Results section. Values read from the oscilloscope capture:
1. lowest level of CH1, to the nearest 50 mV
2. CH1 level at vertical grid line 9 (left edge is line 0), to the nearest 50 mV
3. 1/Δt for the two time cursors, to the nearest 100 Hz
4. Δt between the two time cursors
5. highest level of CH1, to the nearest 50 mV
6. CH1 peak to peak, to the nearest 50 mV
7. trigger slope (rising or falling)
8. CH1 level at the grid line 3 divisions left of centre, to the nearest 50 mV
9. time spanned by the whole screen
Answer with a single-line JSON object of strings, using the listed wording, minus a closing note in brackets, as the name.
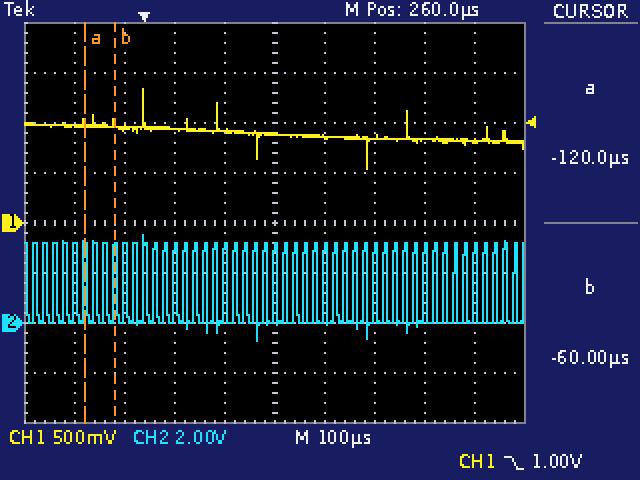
{"lowest level of CH1, to the nearest 50 mV": "550 mV", "CH1 level at vertical grid line 9 (left edge is line 0), to the nearest 50 mV": "800 mV", "1/Δt for the two time cursors, to the nearest 100 Hz": "16.7 kHz", "Δt between the two time cursors": "60 µs", "highest level of CH1, to the nearest 50 mV": "1.35 V", "CH1 peak to peak, to the nearest 50 mV": "800 mV", "trigger slope": "falling", "CH1 level at the grid line 3 divisions left of centre, to the nearest 50 mV": "950 mV", "time spanned by the whole screen": "1 ms"}
